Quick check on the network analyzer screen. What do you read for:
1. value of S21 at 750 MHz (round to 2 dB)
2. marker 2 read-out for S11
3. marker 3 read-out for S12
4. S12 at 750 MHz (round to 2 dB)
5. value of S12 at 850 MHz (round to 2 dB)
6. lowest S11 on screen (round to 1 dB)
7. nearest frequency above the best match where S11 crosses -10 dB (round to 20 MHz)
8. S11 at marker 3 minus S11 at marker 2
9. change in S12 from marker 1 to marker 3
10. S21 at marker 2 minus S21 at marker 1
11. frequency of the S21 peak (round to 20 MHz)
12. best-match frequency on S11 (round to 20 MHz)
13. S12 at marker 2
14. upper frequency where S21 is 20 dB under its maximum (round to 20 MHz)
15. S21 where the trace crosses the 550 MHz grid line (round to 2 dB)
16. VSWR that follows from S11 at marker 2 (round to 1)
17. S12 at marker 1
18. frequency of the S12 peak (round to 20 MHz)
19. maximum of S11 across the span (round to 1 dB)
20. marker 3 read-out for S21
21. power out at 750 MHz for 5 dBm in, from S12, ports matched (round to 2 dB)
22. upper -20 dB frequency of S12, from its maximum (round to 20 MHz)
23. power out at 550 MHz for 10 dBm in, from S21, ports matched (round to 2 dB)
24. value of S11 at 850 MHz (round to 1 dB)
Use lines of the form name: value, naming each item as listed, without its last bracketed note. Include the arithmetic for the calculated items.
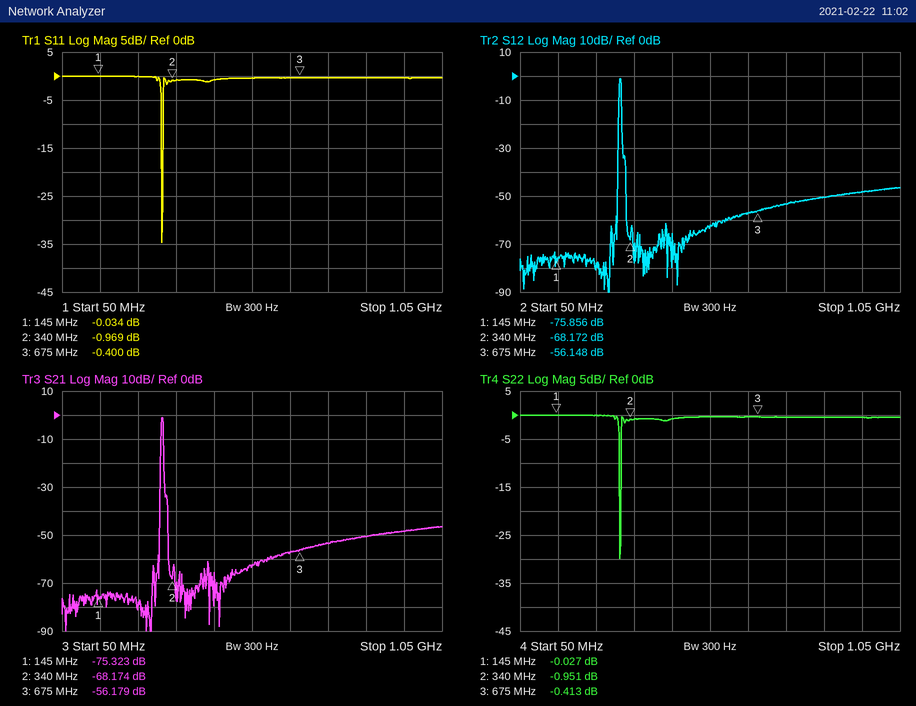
value of S21 at 750 MHz: -54 dB
marker 2 read-out for S11: -0.969 dB
marker 3 read-out for S12: -56.148 dB
S12 at 750 MHz: -54 dB
value of S12 at 850 MHz: -50 dB
lowest S11 on screen: -35 dB
nearest frequency above the best match where S11 crosses -10 dB: 320 MHz
S11 at marker 3 minus S11 at marker 2: -0.4 − (-0.969) = 0.569 dB
change in S12 from marker 1 to marker 3: -56.148 − (-75.856) = 19.708 dB
S21 at marker 2 minus S21 at marker 1: -68.174 − (-75.323) = 7.149 dB
frequency of the S21 peak: 320 MHz
best-match frequency on S11: 320 MHz
S12 at marker 2: -68.172 dB
upper frequency where S21 is 20 dB under its maximum: 320 MHz
S21 where the trace crosses the 550 MHz grid line: -62 dB
VSWR that follows from S11 at marker 2: (1 + 0.8944)/(1 − 0.8944) ≈ 18
S12 at marker 1: -75.856 dB
frequency of the S12 peak: 320 MHz
maximum of S11 across the span: 0 dB
marker 3 read-out for S21: -56.179 dB
power out at 750 MHz for 5 dBm in, from S12, ports matched: 5 dBm + (-54 dB) = -48 dBm
upper -20 dB frequency of S12, from its maximum: 320 MHz
power out at 550 MHz for 10 dBm in, from S21, ports matched: 10 dBm + (-62 dB) = -52 dBm
value of S11 at 850 MHz: 0 dB
